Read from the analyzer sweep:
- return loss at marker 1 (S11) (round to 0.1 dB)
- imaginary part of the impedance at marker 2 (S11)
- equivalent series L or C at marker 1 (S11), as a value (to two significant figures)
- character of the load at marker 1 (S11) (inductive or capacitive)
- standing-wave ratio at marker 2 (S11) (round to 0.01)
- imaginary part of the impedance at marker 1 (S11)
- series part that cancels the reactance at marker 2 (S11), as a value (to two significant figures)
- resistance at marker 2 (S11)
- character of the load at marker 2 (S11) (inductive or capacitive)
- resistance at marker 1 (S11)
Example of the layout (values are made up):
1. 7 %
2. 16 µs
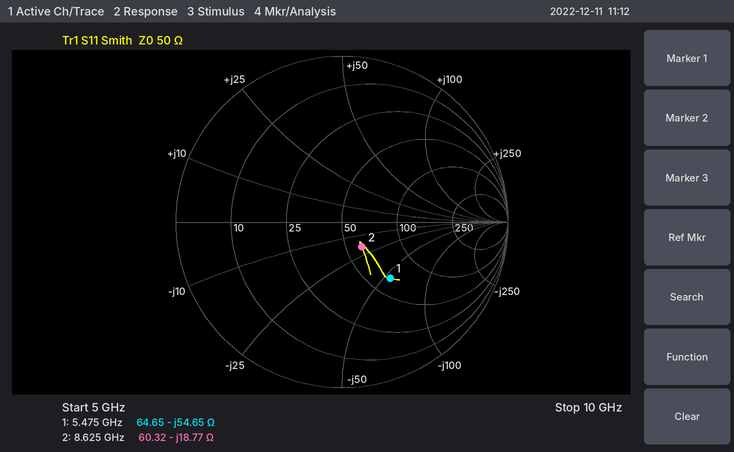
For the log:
1. 7.0 dB
2. -18.77 Ω
3. 530 fF
4. capacitive
5. 1.47
6. -54.65 Ω
7. 350 pH
8. 60.32 Ω
9. capacitive
10. 64.65 Ω
